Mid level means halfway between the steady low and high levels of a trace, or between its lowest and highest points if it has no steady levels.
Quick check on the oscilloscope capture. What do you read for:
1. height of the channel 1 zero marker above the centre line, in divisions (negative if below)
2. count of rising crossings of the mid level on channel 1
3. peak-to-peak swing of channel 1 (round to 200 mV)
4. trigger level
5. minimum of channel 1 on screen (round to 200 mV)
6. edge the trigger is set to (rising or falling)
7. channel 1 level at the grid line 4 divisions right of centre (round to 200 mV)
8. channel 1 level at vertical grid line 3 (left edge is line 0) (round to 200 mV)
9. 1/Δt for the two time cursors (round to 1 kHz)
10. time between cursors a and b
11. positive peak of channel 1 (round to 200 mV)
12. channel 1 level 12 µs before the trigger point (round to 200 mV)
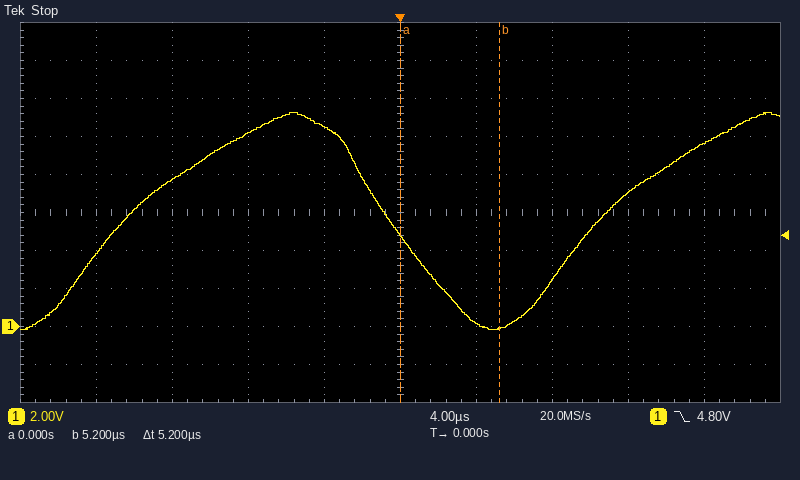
-3.0 div
2
11.4 V
4.80 V
-200 mV
falling
9.6 V
10.2 V
192 kHz
5.2 µs
11.2 V
7.8 V
